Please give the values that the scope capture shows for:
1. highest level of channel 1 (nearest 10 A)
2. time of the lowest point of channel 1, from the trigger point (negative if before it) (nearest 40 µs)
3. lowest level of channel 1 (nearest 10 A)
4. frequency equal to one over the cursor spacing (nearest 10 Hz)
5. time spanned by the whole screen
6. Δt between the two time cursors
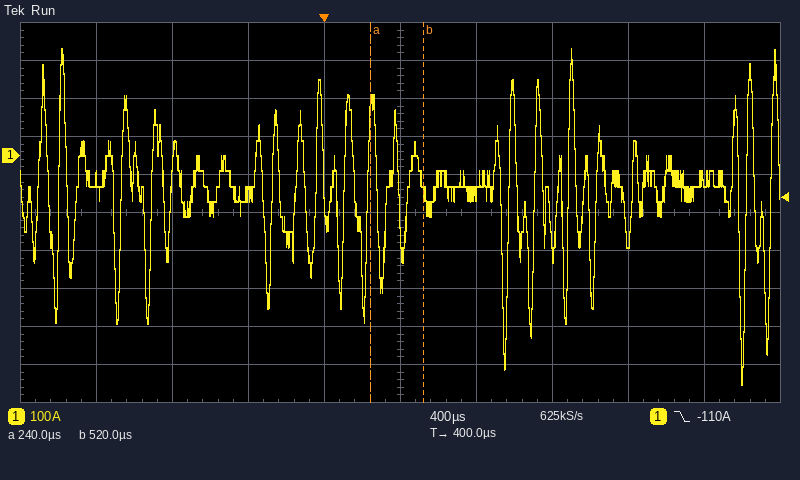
280 A
+2.20 ms
-600 A
3.57 kHz
4 ms
280 µs
